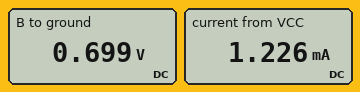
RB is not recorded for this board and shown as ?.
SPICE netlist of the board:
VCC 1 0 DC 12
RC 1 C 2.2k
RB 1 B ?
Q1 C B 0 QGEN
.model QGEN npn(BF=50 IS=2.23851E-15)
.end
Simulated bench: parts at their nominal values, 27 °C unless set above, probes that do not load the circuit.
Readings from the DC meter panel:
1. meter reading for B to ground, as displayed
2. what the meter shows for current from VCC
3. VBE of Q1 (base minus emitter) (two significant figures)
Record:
0.699 V
1.226 mA
700 mV
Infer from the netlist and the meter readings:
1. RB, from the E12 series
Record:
470 kΩ
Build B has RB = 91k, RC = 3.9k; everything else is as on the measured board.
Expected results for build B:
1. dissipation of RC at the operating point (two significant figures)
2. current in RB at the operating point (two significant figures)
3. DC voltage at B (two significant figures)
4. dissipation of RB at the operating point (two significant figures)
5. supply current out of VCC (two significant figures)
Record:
36 mW
120 µA
720 mV
1.4 mW
3.2 mA
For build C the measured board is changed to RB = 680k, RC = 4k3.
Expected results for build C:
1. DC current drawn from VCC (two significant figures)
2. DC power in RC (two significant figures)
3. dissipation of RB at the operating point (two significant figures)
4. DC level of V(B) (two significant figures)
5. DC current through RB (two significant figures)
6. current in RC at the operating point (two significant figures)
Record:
850 µA
3.0 mW
190 µW
690 mV
17 µA
830 µA
